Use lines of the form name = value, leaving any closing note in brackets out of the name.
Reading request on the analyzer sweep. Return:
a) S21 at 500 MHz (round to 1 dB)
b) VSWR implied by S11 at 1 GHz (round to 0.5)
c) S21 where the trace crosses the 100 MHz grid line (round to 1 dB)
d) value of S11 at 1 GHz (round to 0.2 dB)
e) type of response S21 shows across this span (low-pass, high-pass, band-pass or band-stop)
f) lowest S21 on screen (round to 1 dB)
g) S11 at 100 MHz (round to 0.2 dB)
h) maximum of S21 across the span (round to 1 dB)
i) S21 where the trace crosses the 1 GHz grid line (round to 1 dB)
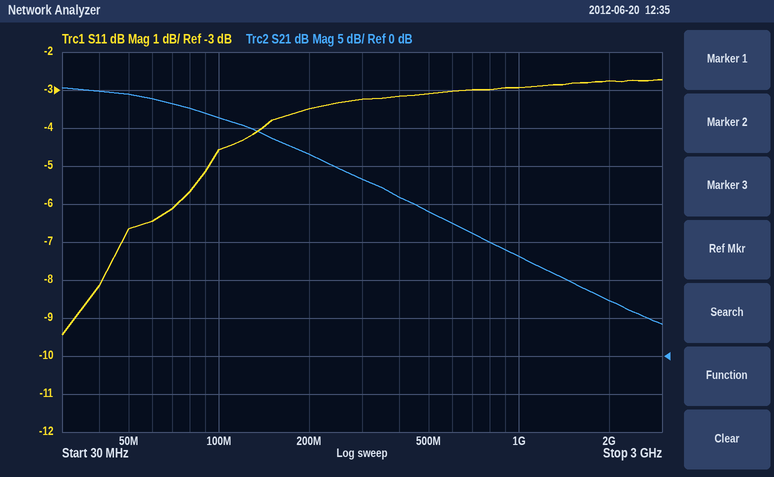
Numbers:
S21 at 500 MHz = 19 dB
VSWR implied by S11 at 1 GHz = 6.0
S21 where the trace crosses the 100 MHz grid line = 31 dB
value of S11 at 1 GHz = -3.0 dB
type of response S21 shows across this span = low-pass
lowest S21 on screen = 4 dB
S11 at 100 MHz = -4.6 dB
maximum of S21 across the span = 35 dB
S21 where the trace crosses the 1 GHz grid line = 13 dB
